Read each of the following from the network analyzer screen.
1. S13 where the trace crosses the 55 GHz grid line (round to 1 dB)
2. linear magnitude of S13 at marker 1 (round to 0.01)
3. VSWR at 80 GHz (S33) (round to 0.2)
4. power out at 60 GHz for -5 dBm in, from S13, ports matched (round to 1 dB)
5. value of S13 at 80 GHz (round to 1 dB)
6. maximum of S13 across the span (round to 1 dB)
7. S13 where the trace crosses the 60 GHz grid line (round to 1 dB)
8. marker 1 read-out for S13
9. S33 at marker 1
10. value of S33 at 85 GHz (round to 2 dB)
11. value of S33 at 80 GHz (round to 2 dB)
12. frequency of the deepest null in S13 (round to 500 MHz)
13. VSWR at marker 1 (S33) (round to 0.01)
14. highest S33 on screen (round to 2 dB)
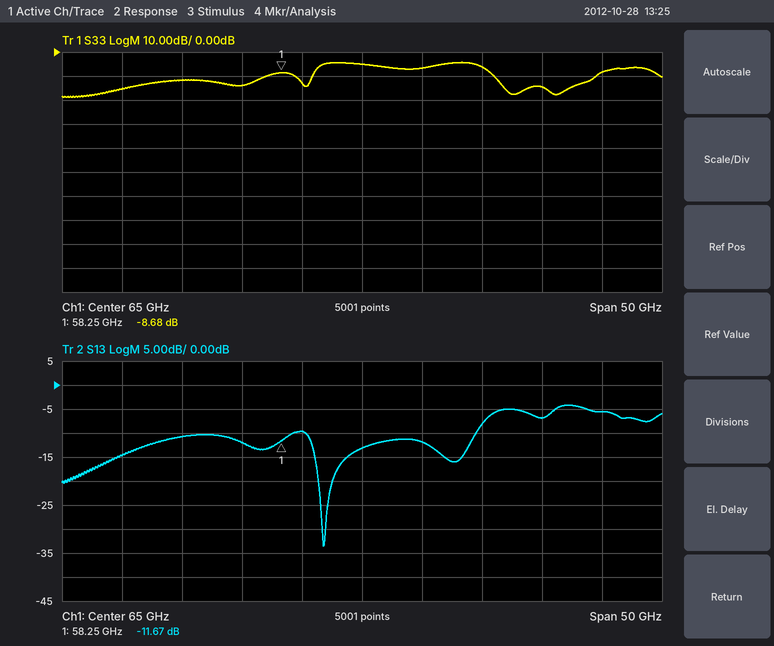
-12 dB
0.26
1.4
-15 dBm
-7 dB
-4 dB
-10 dB
-11.67 dB
-8.68 dB
-8 dB
-14 dB
62.0 GHz
2.17
-4 dB
